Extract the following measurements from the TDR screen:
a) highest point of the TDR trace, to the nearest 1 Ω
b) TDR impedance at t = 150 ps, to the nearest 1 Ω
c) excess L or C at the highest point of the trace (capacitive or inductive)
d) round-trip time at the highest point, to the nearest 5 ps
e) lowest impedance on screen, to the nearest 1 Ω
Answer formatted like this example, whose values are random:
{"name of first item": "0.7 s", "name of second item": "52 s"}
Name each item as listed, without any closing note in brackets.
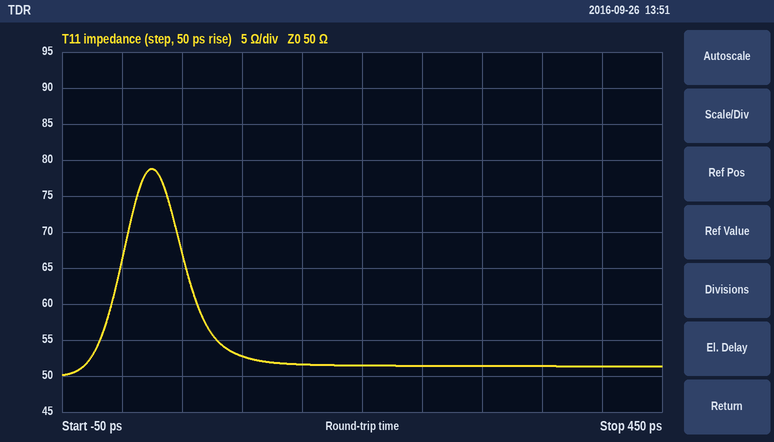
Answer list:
{"highest point of the TDR trace, to the nearest 1 Ω": "79 Ω", "TDR impedance at t = 150 ps, to the nearest 1 Ω": "52 Ω", "excess L or C at the highest point of the trace": "inductive", "round-trip time at the highest point, to the nearest 5 ps": "25 ps", "lowest impedance on screen, to the nearest 1 Ω": "50 Ω"}
